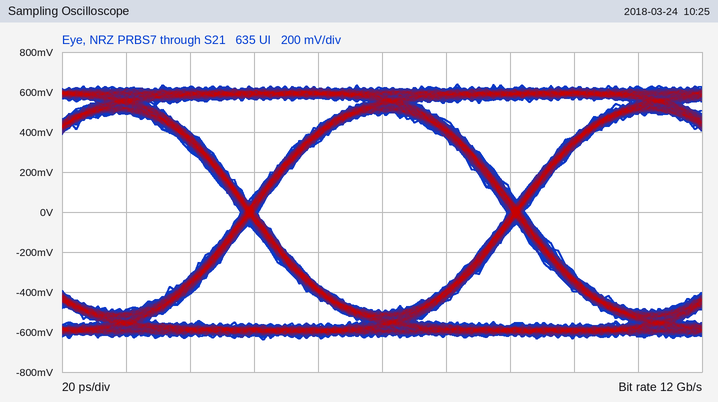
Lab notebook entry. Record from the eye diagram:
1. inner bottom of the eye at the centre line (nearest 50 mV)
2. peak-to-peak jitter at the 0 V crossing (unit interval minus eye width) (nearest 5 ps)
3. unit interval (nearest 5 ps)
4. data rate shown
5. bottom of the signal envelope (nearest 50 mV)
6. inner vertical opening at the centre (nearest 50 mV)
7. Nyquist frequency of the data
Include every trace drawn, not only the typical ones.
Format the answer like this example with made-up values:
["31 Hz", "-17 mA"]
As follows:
["-500 mV", "5 ps", "85 ps", "12 Gb/s", "-650 mV", "1.00 V", "6 GHz"]
